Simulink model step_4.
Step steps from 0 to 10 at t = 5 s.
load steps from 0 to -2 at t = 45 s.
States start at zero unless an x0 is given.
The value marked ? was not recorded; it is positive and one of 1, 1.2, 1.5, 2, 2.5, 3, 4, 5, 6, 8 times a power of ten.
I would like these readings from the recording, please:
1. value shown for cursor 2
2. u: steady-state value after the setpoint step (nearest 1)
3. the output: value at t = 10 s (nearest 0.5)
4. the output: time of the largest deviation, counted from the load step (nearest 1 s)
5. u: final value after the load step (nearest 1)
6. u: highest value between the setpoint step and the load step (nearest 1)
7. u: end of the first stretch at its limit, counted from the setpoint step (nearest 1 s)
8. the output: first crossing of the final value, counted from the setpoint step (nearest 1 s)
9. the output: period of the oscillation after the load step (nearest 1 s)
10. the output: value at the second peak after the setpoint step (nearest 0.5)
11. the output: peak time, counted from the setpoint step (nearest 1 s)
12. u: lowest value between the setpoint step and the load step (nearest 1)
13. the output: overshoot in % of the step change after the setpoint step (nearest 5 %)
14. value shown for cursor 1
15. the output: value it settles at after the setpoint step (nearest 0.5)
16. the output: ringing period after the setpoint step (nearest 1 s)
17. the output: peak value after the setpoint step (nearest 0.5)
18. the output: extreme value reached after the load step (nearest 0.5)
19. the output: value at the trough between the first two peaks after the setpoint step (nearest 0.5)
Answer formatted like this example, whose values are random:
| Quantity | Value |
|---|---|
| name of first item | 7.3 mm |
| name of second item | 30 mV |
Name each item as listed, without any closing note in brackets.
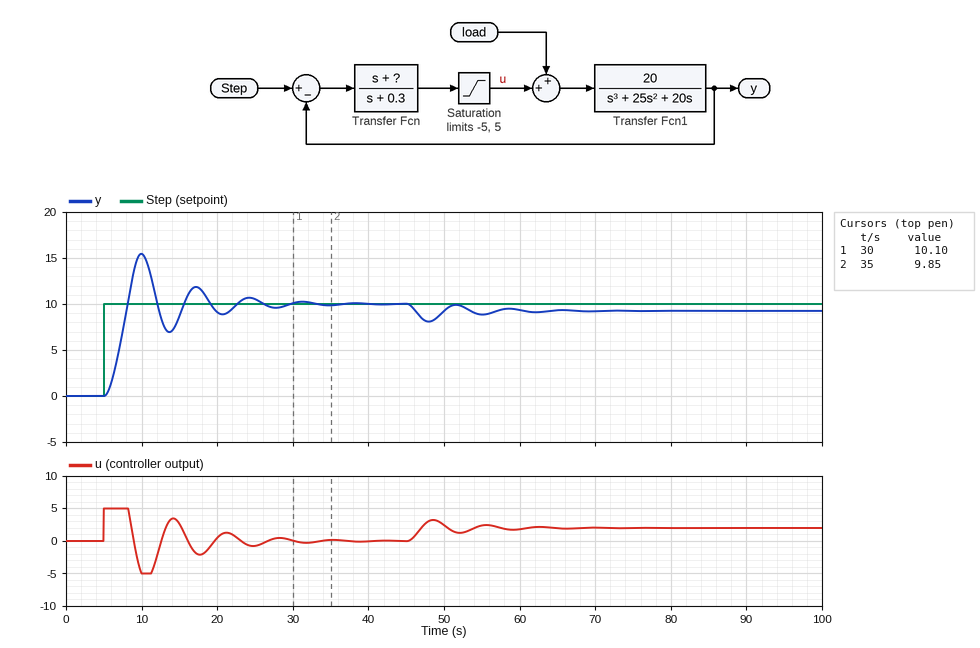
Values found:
| Quantity | Value |
|---|---|
| value shown for cursor 2 | 9.85 |
| u: steady-state value after the setpoint step | 0 |
| the output: value at t = 10 s | 15.5 |
| the output: time of the largest deviation, counted from the load step | 3 s |
| u: final value after the load step | 2 |
| u: highest value between the setpoint step and the load step | 5 |
| u: end of the first stretch at its limit, counted from the setpoint step | 3 s |
| the output: first crossing of the final value, counted from the setpoint step | 3 s |
| the output: period of the oscillation after the load step | 7 s |
| the output: value at the second peak after the setpoint step | 12.0 |
| the output: peak time, counted from the setpoint step | 5 s |
| u: lowest value between the setpoint step and the load step | -5 |
| the output: overshoot in % of the step change after the setpoint step | 55 % |
| value shown for cursor 1 | 10.10 |
| the output: value it settles at after the setpoint step | 10.0 |
| the output: ringing period after the setpoint step | 7 s |
| the output: peak value after the setpoint step | 15.5 |
| the output: extreme value reached after the load step | 8.0 |
| the output: value at the trough between the first two peaks after the setpoint step | 7.0 |
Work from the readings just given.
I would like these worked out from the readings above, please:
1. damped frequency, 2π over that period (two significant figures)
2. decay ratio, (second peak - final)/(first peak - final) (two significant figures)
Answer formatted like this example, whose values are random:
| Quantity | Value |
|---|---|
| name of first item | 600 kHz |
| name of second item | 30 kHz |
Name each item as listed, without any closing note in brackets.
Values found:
| Quantity | Value |
|---|---|
| damped frequency, 2π over that period | 0.90 rad/s |
| decay ratio, (second peak - final)/(first peak - final) | 0.36 |
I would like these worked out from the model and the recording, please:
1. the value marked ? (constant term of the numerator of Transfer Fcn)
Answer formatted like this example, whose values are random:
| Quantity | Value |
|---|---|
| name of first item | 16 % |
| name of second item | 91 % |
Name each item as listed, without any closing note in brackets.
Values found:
| Quantity | Value |
|---|---|
| the value marked ? | 0.8 |
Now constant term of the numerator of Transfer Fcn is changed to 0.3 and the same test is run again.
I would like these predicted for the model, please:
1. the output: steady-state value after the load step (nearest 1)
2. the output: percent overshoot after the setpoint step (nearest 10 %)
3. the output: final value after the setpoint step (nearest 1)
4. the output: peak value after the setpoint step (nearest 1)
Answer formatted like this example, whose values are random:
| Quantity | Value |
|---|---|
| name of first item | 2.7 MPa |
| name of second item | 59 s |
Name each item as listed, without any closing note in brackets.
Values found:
| Quantity | Value |
|---|---|
| the output: steady-state value after the load step | 8 |
| the output: percent overshoot after the setpoint step | 20 % |
| the output: final value after the setpoint step | 10 |
| the output: peak value after the setpoint step | 12 |
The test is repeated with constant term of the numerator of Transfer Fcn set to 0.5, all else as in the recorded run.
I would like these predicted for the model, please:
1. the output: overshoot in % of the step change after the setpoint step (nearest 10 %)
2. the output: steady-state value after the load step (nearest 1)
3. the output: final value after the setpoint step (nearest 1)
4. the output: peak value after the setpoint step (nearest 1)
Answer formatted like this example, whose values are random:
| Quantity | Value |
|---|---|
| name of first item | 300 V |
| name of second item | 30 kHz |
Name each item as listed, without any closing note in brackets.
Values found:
| Quantity | Value |
|---|---|
| the output: overshoot in % of the step change after the setpoint step | 40 % |
| the output: steady-state value after the load step | 9 |
| the output: final value after the setpoint step | 10 |
| the output: peak value after the setpoint step | 14 |
